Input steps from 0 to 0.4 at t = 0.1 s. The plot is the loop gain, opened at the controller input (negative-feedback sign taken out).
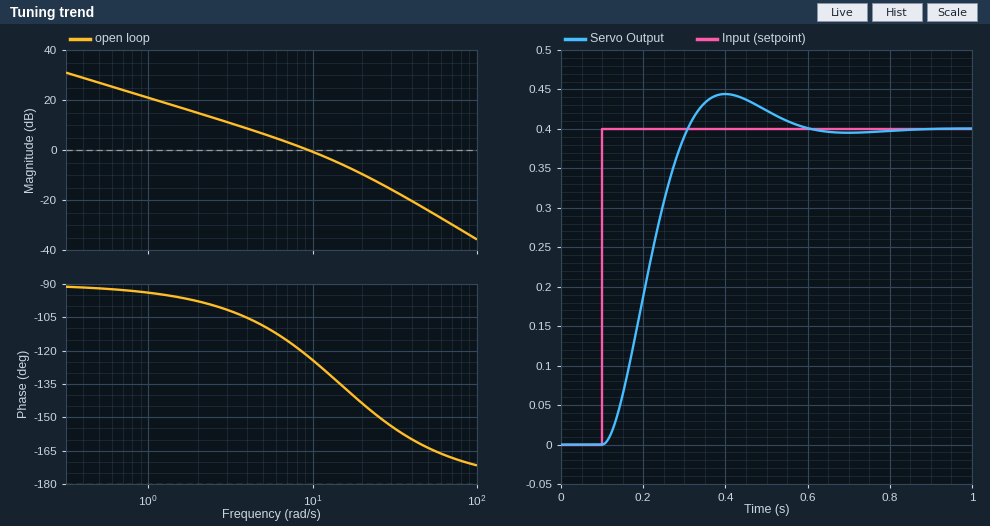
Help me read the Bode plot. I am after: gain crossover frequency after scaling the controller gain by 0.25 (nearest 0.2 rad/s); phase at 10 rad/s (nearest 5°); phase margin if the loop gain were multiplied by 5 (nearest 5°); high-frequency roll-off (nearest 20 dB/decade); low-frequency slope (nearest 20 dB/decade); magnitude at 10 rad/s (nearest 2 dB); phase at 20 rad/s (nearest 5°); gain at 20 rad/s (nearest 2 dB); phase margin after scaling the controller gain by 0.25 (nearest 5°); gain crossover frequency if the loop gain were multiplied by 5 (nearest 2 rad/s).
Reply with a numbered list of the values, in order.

1. 2.8 rad/s
2. -125°
3. 30°
4. -40 dB/decade
5. -20 dB/decade
6. 0 dB
7. -145°
8. -10 dB
9. 80°
10. 26 rad/s
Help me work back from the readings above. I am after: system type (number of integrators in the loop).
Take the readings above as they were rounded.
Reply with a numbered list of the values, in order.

1. 1
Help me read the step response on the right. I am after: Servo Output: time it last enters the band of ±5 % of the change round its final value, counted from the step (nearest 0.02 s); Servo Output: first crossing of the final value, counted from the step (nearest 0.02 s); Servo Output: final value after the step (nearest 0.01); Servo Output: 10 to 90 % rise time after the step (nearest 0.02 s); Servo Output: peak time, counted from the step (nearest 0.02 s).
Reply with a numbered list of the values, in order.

1. 0.42 s
2. 0.20 s
3. 0.40
4. 0.14 s
5. 0.30 s
